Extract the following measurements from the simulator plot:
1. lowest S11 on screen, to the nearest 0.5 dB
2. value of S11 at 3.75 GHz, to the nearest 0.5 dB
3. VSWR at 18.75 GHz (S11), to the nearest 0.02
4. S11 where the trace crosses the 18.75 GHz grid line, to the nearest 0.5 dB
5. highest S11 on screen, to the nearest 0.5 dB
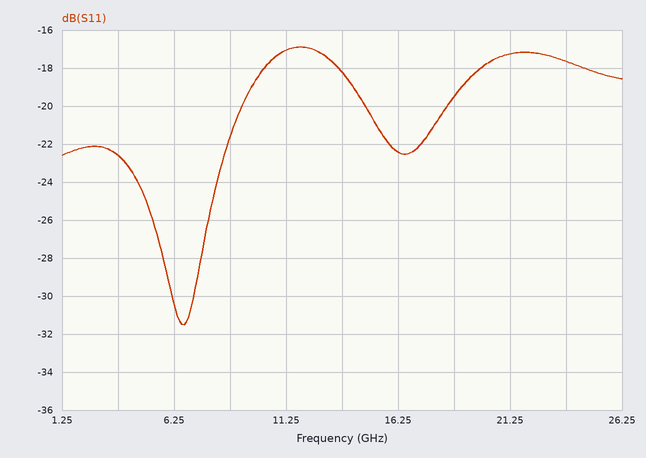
-31.5 dB
-22.5 dB
1.24
-19.5 dB
-17.0 dB
